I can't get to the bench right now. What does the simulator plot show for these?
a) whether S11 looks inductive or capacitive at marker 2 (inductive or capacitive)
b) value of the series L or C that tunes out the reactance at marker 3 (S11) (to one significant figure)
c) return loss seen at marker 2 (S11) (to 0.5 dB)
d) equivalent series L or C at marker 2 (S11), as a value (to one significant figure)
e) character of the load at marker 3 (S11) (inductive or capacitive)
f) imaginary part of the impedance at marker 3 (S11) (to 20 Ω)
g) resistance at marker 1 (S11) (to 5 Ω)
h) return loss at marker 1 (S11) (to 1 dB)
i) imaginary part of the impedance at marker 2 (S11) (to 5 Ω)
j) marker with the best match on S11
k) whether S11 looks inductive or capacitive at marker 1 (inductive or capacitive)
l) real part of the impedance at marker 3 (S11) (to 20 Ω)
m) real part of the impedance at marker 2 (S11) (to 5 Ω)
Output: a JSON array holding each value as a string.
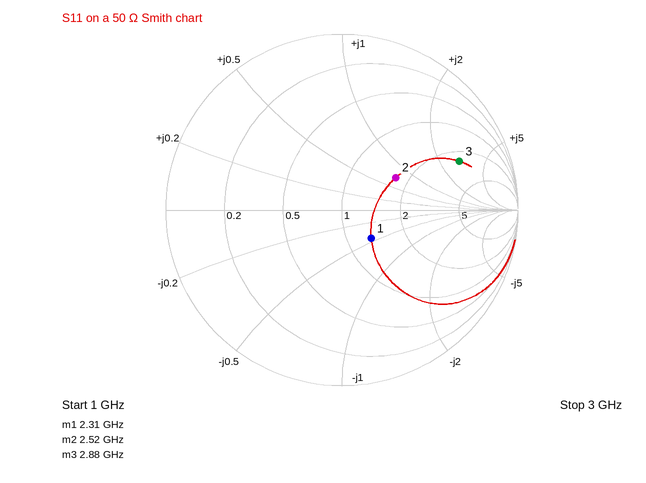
["inductive", "400 fF", "9.0 dB", "2 nH", "inductive", "+140 Ω", "65 Ω", "13 dB", "+35 Ω", "marker 1", "capacitive", "120 Ω", "85 Ω"]
